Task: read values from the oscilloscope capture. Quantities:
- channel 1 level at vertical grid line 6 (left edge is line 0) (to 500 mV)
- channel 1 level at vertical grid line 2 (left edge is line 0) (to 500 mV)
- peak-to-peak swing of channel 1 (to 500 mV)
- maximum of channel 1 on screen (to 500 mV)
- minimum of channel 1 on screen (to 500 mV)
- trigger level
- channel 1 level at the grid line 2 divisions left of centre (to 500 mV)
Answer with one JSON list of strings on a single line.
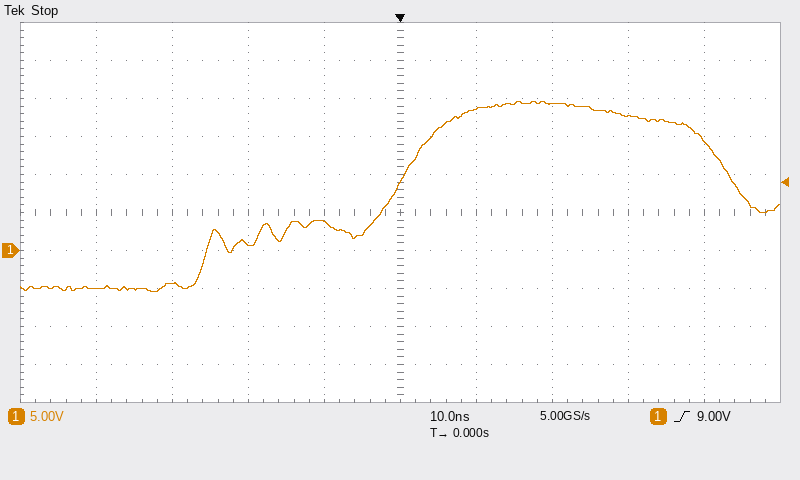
["18.5 V", "-4.5 V", "25.0 V", "19.5 V", "-5.5 V", "9.00 V", "1.0 V"]
